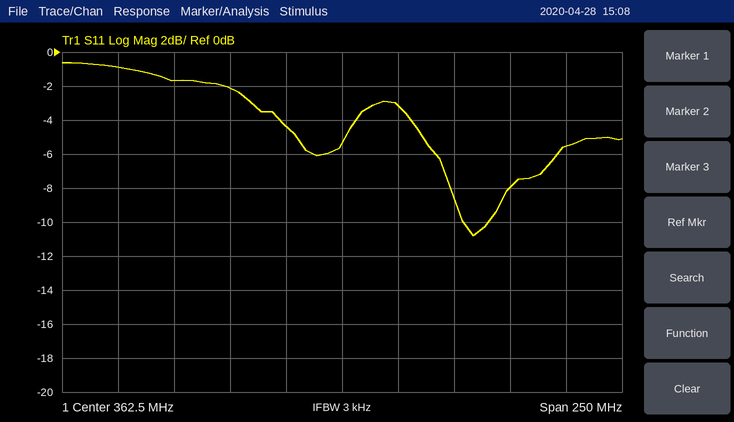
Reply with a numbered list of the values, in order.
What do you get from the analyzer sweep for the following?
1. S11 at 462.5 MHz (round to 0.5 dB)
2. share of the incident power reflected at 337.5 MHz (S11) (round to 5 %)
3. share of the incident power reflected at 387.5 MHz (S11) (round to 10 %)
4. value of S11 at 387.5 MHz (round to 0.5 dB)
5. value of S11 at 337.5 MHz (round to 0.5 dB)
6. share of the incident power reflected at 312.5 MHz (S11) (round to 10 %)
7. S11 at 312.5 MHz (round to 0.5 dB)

1. -5.5 dB
2. 35 %
3. 50 %
4. -3.0 dB
5. -4.5 dB
6. 60 %
7. -2.0 dB
